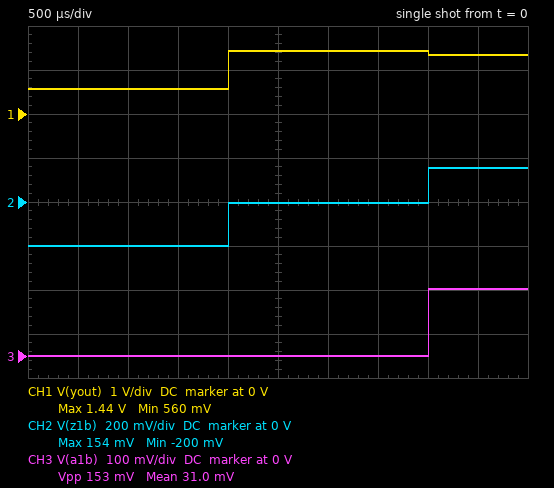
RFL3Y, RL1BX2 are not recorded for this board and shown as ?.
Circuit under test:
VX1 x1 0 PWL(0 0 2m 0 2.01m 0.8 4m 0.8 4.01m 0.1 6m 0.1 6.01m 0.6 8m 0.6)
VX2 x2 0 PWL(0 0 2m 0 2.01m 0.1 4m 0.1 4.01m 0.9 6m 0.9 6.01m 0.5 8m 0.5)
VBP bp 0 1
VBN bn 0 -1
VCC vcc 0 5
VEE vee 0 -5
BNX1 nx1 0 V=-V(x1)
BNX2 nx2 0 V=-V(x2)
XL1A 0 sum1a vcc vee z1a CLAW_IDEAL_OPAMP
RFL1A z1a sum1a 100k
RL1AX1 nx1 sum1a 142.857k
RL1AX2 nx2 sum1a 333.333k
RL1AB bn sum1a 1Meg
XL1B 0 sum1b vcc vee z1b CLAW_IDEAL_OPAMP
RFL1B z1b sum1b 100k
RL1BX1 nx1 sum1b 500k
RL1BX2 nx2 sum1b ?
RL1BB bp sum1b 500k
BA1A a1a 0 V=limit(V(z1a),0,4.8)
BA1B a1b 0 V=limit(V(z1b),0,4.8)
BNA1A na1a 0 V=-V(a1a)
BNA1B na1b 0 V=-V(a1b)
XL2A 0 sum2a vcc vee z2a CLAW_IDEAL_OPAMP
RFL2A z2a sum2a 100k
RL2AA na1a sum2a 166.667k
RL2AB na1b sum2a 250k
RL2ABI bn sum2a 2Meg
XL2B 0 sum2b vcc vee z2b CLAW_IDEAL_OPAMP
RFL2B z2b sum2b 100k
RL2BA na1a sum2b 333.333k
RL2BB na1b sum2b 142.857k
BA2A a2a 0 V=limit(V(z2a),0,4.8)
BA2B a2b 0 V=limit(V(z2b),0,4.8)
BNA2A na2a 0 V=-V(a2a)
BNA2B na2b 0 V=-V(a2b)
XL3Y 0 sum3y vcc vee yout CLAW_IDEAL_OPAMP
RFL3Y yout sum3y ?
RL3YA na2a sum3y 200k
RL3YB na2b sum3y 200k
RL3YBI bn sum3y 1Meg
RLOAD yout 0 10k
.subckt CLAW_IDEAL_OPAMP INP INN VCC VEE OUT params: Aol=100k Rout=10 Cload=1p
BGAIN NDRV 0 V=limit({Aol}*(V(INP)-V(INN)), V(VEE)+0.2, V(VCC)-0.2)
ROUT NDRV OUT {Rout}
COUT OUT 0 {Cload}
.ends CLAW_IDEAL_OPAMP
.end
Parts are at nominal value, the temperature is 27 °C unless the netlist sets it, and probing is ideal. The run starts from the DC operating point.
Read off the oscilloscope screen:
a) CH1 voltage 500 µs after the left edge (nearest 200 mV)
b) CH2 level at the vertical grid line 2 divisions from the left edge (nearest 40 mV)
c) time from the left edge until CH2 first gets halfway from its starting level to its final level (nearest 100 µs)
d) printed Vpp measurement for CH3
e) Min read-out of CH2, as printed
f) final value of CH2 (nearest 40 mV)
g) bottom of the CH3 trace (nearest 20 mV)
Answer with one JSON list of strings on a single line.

["600 mV", "-200 mV", "2.0 ms", "153 mV", "-200 mV", "160 mV", "0 V"]
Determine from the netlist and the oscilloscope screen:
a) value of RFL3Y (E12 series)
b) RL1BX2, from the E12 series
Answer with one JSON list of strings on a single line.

["330 kΩ", "270 kΩ"]
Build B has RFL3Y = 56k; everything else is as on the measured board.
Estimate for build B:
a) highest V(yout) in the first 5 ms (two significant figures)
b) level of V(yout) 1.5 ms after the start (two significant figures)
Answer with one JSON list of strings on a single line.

["240 mV", "95 mV"]
